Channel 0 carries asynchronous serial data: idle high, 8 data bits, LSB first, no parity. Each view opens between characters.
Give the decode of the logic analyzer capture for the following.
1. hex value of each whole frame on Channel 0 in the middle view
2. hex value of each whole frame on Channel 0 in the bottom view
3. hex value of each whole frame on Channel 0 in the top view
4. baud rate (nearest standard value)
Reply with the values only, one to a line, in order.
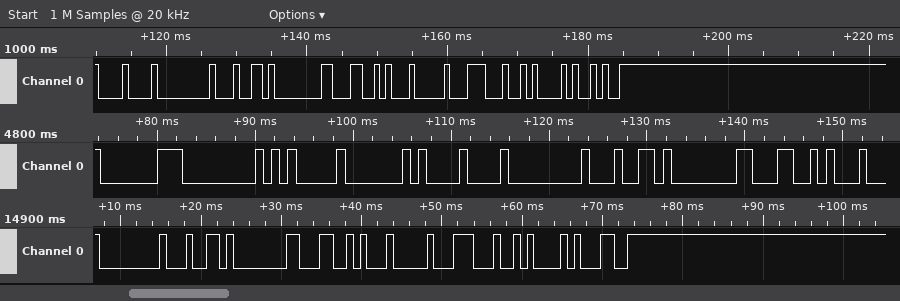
C0, 00, 05, 40, 08, 00, 64, 80, 4C
00, 64, 80, 4C, 04, 1C, 0A, 31
08, 00, 64, 80, 4C, 04, 1C, 0A, 29
1200 baud
